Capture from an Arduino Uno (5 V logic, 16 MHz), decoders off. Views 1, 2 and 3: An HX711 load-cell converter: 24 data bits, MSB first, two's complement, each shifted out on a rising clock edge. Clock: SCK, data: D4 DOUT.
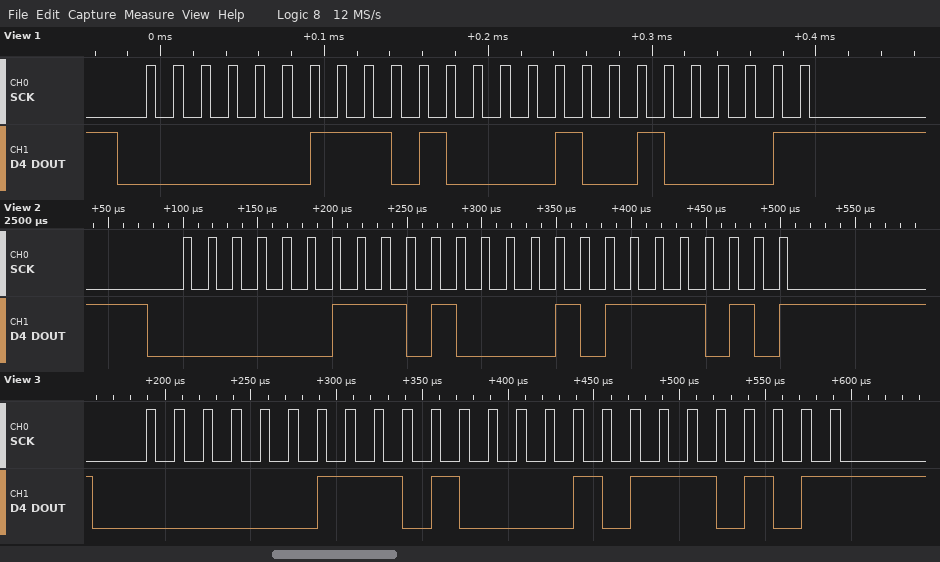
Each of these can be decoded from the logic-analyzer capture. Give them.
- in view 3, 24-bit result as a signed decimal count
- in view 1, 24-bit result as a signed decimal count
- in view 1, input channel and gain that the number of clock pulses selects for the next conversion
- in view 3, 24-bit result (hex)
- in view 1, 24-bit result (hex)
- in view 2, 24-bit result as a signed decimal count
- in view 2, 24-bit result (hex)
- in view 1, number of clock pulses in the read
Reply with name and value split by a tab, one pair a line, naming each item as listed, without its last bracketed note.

in view 3, 24-bit result as a signed decimal count	237941
in view 1, 24-bit result as a signed decimal count	237857
in view 1, input channel and gain that the number of clock pulses selects for the next conversion	channel A, gain 128
in view 3, 24-bit result	0x03A175
in view 1, 24-bit result	0x03A121
in view 2, 24-bit result as a signed decimal count	237946
in view 2, 24-bit result	0x03A17A
in view 1, number of clock pulses in the read	25
